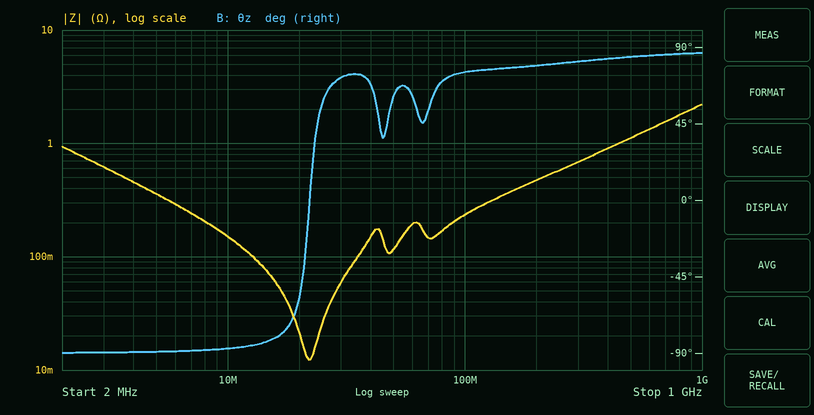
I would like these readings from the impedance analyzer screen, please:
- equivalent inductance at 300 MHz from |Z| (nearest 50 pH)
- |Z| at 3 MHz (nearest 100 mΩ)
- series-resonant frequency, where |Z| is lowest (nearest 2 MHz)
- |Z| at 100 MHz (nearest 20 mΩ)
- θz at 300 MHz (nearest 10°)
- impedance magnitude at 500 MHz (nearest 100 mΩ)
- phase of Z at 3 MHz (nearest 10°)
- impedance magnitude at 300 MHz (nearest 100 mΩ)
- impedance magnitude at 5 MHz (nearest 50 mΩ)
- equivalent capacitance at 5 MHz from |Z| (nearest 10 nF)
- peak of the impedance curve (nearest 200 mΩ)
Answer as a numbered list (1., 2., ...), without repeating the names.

1. 350 pH
2. 600 mΩ
3. 22 MHz
4. 240 mΩ
5. 80°
6. 1.1 Ω
7. -90°
8. 700 mΩ
9. 350 mΩ
10. 90 nF
11. 2.2 Ω
